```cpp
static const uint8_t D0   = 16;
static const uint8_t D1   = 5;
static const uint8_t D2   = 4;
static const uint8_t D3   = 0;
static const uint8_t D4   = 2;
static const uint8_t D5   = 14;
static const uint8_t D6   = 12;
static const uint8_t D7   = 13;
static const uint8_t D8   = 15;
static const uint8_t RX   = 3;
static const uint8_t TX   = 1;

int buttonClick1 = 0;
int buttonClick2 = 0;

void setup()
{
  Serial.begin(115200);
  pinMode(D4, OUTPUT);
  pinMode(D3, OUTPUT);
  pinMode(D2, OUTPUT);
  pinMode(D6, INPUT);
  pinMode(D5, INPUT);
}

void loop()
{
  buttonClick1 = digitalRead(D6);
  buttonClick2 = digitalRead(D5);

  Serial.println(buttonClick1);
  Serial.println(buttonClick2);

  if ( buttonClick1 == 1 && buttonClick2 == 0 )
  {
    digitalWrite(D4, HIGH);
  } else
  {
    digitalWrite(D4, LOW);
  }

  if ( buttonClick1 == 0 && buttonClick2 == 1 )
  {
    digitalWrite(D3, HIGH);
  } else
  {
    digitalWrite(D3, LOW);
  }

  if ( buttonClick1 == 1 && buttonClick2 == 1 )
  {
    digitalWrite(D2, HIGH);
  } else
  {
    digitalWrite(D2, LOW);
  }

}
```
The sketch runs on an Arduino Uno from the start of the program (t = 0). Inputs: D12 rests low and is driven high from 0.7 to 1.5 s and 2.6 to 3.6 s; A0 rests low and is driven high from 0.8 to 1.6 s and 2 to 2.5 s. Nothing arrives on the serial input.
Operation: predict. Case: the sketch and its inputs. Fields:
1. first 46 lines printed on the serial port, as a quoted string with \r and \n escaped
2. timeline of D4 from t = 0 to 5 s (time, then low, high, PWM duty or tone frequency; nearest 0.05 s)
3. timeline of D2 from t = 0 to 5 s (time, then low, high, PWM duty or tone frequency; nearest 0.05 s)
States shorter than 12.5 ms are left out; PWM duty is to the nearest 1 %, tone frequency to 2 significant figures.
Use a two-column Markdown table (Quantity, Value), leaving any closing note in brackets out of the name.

| Quantity | Value |
|---|---|
| first 46 lines printed on the serial port, as a quoted string with \r and \n escaped | "0\r\n0\r\n0\r\n0\r\n0\r\n0\r\n0\r\n0\r\n0\r\n0\r\n0\r\n0\r\n0\r\n0\r\n0\r\n0\r\n0\r\n0\r\n0\r\n0\r\n0\r\n0\r\n0\r\n0\r\n0\r\n0\r\n0\r\n0\r\n0\r\n0\r\n0\r\n0\r\n0\r\n0\r\n0\r\n0\r\n0\r\n0\r\n0\r\n0\r\n0\r\n0\r\n0\r\n0\r\n0\r\n0\r\n" |
| timeline of D4 from t = 0 to 5 s | 0 s low; 0.8 s high; 1.5 s low |
| timeline of D2 from t = 0 to 5 s | 0 s low; 0.7 s high; 0.8 s low; 2.6 s high; 3.6 s low |
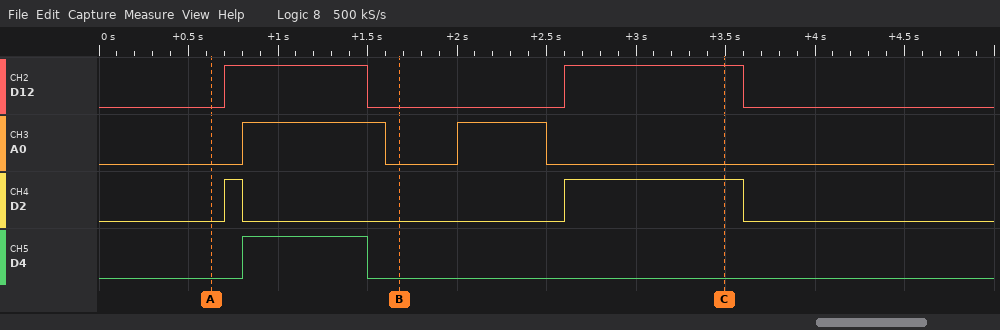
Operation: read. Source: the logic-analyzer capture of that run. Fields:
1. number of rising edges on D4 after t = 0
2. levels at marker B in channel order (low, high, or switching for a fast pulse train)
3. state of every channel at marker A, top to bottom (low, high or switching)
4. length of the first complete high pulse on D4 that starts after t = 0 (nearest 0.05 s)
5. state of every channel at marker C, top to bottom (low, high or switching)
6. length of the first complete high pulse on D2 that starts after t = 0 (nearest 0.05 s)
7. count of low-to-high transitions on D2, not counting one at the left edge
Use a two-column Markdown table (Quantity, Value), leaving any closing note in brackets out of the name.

| Quantity | Value |
|---|---|
| number of rising edges on D4 after t = 0 | 1 |
| levels at marker B in channel order | D12 low, A0 low, D2 low, D4 low |
| state of every channel at marker A, top to bottom | D12 low, A0 low, D2 low, D4 low |
| length of the first complete high pulse on D4 that starts after t = 0 | 0.70 s |
| state of every channel at marker C, top to bottom | D12 high, A0 low, D2 high, D4 low |
| length of the first complete high pulse on D2 that starts after t = 0 | 0.10 s |
| count of low-to-high transitions on D2, not counting one at the left edge | 2 |
